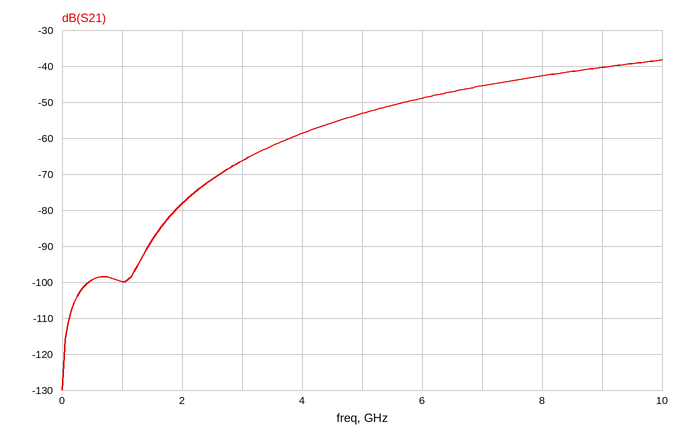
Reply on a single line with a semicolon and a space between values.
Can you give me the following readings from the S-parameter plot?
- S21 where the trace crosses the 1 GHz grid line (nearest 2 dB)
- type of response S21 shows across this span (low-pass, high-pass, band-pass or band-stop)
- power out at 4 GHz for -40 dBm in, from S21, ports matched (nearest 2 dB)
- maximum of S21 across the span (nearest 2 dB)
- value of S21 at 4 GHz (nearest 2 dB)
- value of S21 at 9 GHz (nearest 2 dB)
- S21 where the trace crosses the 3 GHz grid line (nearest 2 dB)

-100 dB; high-pass; -98 dBm; -38 dB; -58 dB; -40 dB; -66 dB
